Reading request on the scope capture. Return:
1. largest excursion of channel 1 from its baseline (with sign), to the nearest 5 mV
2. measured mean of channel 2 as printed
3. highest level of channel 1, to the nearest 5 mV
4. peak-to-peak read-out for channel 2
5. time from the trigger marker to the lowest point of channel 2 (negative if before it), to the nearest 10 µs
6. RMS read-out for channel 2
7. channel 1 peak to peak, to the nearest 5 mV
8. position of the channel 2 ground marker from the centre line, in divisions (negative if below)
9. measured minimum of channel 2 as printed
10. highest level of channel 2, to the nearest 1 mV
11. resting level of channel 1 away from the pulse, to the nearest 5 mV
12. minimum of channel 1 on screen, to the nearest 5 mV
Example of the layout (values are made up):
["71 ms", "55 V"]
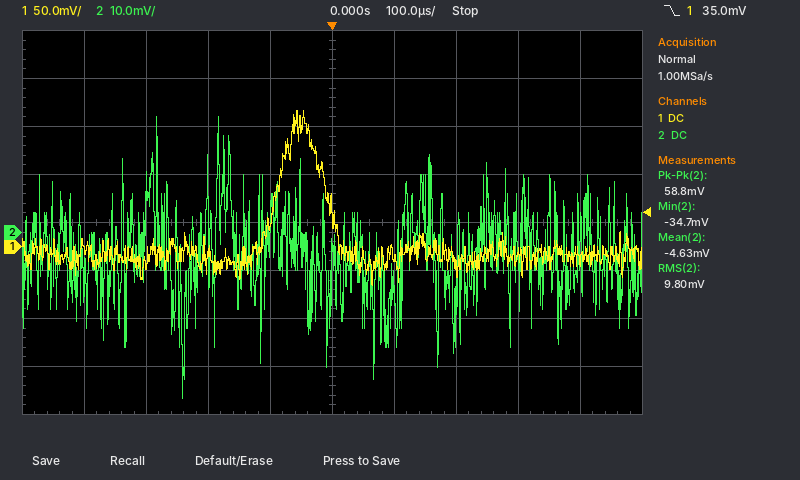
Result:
["+150 mV", "-4.63 mV", "140 mV", "58.8 mV", "-240 µs", "9.80 mV", "180 mV", "-0.2 div", "-34.7 mV", "24 mV", "-10 mV", "-40 mV"]
